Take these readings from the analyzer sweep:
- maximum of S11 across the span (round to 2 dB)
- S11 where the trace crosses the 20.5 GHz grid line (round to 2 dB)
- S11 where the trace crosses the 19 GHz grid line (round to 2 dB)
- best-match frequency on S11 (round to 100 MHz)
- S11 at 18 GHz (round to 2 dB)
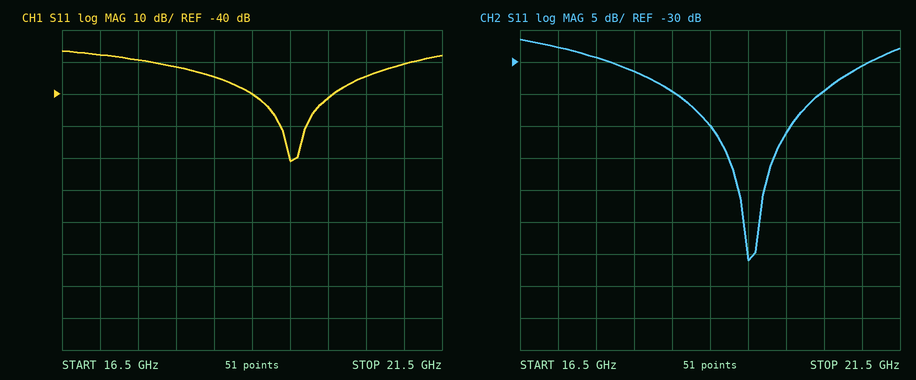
-26 dB
-34 dB
-40 dB
19.5 GHz
-32 dB
